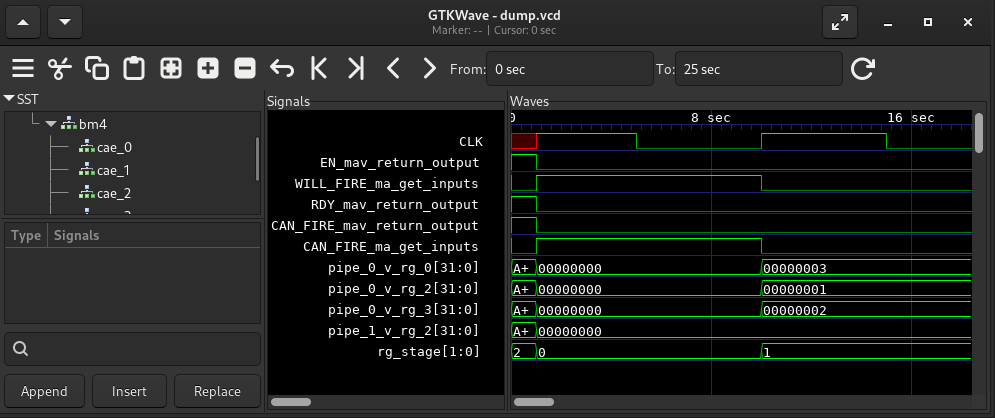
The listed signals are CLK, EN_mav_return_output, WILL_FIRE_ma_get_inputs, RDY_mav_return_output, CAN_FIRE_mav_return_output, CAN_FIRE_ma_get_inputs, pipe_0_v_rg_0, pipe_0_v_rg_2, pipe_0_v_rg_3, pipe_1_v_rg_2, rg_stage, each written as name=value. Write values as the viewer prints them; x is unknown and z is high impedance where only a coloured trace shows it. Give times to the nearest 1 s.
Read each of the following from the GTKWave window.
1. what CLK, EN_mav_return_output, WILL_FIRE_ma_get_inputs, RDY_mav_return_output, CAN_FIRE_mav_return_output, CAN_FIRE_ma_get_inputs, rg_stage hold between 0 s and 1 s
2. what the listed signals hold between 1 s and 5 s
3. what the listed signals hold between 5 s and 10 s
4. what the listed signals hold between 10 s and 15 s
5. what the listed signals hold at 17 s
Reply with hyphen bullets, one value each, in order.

- CLK=x, EN_mav_return_output=1, WILL_FIRE_ma_get_inputs=0, RDY_mav_return_output=1, CAN_FIRE_mav_return_output=1, CAN_FIRE_ma_get_inputs=0, rg_stage=2
- CLK=1, EN_mav_return_output=0, WILL_FIRE_ma_get_inputs=1, RDY_mav_return_output=0, CAN_FIRE_mav_return_output=0, CAN_FIRE_ma_get_inputs=1, pipe_0_v_rg_0=00000000, pipe_0_v_rg_2=00000000, pipe_0_v_rg_3=00000000, pipe_1_v_rg_2=00000000, rg_stage=0
- CLK=0, EN_mav_return_output=0, WILL_FIRE_ma_get_inputs=1, RDY_mav_return_output=0, CAN_FIRE_mav_return_output=0, CAN_FIRE_ma_get_inputs=1, pipe_0_v_rg_0=00000000, pipe_0_v_rg_2=00000000, pipe_0_v_rg_3=00000000, pipe_1_v_rg_2=00000000, rg_stage=0
- CLK=1, EN_mav_return_output=0, WILL_FIRE_ma_get_inputs=0, RDY_mav_return_output=0, CAN_FIRE_mav_return_output=0, CAN_FIRE_ma_get_inputs=0, pipe_0_v_rg_0=00000003, pipe_0_v_rg_2=00000001, pipe_0_v_rg_3=00000002, pipe_1_v_rg_2=00000000, rg_stage=1
- CLK=0, EN_mav_return_output=0, WILL_FIRE_ma_get_inputs=0, RDY_mav_return_output=0, CAN_FIRE_mav_return_output=0, CAN_FIRE_ma_get_inputs=0, pipe_0_v_rg_0=00000003, pipe_0_v_rg_2=00000001, pipe_0_v_rg_3=00000002, pipe_1_v_rg_2=00000000, rg_stage=1
